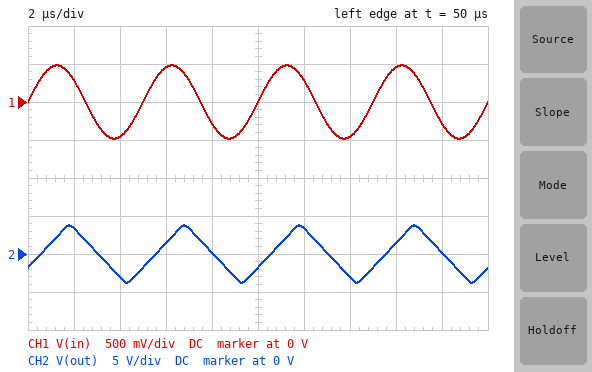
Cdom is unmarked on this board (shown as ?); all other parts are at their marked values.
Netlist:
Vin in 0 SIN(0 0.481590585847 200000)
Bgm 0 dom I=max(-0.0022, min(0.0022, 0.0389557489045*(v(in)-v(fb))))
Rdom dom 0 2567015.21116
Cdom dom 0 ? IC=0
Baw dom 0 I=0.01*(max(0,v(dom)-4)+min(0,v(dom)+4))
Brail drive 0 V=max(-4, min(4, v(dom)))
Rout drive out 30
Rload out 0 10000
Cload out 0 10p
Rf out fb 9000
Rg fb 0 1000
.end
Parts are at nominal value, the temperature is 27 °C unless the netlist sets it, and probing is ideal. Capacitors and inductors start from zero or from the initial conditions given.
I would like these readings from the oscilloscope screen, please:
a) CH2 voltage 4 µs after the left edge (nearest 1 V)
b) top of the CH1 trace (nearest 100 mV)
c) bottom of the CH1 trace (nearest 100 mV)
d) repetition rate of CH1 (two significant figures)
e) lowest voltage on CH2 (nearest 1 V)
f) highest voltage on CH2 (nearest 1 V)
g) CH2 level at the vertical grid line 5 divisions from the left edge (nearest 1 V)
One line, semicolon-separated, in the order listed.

-3 V; 500 mV; -500 mV; 200 kHz; -4 V; 4 V; -2 V
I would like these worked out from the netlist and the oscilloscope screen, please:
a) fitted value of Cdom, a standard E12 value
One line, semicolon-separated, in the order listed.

680 pF
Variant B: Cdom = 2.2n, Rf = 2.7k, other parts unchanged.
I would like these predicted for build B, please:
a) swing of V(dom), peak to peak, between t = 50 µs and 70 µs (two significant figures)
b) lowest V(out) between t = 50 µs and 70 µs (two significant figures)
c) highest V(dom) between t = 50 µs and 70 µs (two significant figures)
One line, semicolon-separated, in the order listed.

2.4 V; -1.2 V; 1.2 V
